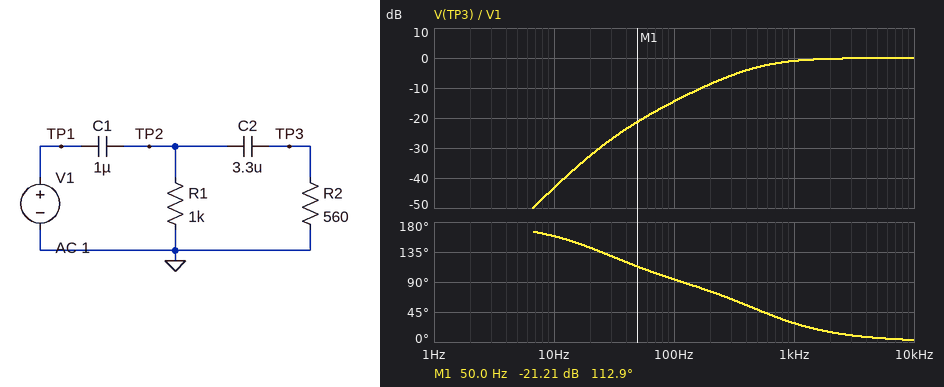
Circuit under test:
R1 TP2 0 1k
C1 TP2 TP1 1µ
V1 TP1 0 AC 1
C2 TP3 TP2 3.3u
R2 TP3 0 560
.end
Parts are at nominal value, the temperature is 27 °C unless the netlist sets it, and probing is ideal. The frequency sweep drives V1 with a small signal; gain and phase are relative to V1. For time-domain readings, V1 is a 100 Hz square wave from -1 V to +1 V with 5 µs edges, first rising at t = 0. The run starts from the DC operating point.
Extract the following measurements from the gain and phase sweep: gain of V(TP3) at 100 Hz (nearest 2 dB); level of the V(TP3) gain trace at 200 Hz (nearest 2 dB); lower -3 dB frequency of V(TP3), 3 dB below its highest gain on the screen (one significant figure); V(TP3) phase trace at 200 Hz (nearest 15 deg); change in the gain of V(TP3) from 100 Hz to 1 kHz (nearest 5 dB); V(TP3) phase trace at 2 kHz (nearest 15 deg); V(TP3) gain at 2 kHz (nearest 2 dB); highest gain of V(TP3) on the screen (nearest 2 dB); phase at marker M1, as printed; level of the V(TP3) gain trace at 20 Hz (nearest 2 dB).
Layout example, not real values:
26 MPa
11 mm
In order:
-14 dB
-8 dB
500 Hz
75 deg
15 dB
15 deg
0 dB
0 dB
112.9 deg
-32 dB
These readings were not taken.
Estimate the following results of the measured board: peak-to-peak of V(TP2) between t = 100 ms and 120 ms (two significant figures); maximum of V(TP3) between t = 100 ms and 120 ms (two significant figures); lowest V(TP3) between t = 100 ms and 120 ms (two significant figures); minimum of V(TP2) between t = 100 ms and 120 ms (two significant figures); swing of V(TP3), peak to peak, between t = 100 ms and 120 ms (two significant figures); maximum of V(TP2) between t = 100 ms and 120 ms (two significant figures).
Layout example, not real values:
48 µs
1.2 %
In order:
3.8 V
2.0 V
-2.0 V
-1.9 V
4.0 V
1.9 V
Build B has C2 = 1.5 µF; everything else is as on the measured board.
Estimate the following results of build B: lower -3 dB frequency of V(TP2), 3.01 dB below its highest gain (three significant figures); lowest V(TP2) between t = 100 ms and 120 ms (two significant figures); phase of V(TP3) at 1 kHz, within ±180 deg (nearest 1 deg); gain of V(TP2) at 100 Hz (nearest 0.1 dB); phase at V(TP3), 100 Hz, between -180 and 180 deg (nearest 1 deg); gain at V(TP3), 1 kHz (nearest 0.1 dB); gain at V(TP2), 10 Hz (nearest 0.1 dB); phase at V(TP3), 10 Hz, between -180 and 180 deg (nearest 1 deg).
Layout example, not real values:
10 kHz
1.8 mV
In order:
521 Hz
-1.9 V
33 deg
-9.8 dB
108 deg
-1.3 dB
-24.2 dB
168 deg
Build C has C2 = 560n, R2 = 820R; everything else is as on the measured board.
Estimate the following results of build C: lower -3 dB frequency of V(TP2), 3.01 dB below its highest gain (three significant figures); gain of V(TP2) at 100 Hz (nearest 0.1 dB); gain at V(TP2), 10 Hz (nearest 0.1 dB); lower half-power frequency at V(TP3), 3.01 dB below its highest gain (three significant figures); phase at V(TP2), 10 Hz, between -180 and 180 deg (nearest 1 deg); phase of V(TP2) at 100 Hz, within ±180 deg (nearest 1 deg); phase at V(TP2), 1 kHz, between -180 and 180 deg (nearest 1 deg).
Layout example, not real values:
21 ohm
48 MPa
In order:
398 Hz
-7.3 dB
-24.1 dB
622 Hz
84 deg
49 deg
17 deg
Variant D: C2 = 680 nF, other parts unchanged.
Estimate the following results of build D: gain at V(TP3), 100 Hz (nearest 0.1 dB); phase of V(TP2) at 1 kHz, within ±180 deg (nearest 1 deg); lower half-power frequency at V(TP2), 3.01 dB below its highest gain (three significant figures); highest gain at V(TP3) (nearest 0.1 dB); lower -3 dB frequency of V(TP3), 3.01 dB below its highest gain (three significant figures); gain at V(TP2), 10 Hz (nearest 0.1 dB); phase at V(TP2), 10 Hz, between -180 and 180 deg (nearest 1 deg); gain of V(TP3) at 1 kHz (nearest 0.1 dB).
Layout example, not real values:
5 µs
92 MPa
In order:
-20.3 dB
20 deg
525 Hz
0 dB
785 Hz
-24.1 dB
84 deg
-2.1 dB
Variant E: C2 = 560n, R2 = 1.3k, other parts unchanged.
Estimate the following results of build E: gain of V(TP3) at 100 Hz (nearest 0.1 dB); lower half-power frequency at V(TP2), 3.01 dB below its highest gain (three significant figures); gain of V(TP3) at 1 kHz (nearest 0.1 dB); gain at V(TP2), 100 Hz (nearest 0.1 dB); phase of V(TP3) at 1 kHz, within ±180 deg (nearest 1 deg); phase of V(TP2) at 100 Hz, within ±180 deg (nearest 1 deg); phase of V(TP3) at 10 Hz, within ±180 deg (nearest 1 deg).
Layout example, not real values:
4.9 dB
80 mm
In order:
-14.9 dB
312 Hz
-0.7 dB
-7.3 dB
27 deg
51 deg
172 deg
